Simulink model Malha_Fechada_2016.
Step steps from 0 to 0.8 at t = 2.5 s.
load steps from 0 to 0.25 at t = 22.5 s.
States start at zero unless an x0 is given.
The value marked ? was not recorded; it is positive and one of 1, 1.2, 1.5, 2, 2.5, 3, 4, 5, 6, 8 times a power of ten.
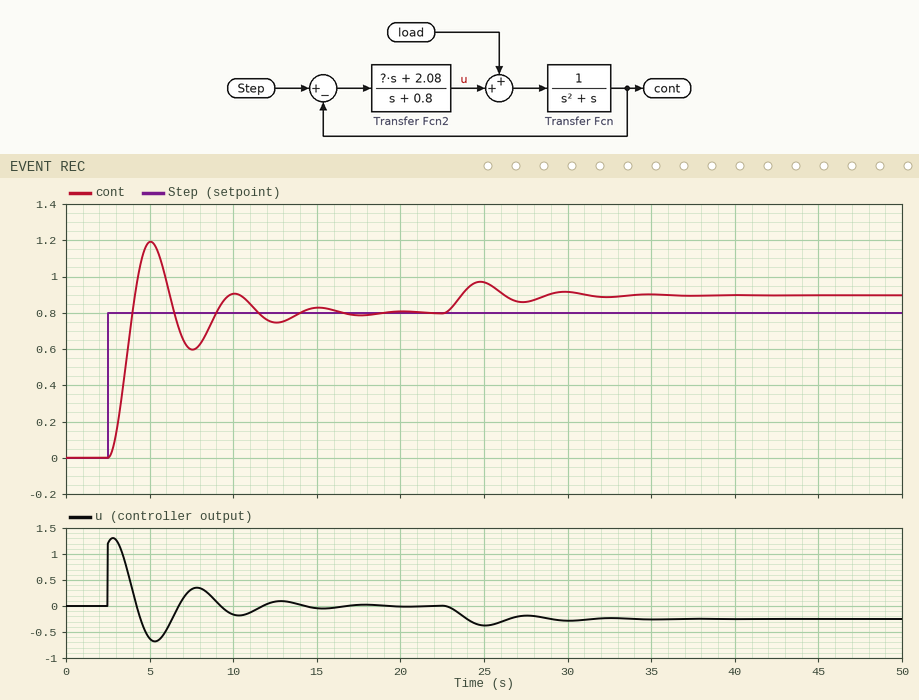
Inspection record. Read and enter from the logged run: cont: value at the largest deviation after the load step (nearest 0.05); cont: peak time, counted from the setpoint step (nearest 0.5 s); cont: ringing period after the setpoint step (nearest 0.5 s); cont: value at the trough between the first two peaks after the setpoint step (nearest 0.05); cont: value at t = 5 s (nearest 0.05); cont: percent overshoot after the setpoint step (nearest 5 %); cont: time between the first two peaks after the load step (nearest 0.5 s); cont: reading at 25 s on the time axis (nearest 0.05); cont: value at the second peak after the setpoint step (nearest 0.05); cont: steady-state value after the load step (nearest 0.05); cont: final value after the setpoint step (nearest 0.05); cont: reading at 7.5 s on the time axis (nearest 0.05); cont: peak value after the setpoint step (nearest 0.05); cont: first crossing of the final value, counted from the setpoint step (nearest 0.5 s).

0.95
2.5 s
5.0 s
0.60
1.20
50 %
5.0 s
0.95
0.90
0.90
0.80
0.60
1.20
1.5 s
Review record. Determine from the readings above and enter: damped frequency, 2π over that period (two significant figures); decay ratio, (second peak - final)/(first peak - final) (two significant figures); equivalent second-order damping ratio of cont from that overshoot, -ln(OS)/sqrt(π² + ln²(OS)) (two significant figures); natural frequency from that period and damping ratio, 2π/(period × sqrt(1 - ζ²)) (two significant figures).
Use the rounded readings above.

1.3 rad/s
0.25
0.22
1.3 rad/s
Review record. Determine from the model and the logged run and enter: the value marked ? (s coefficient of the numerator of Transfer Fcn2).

1.5
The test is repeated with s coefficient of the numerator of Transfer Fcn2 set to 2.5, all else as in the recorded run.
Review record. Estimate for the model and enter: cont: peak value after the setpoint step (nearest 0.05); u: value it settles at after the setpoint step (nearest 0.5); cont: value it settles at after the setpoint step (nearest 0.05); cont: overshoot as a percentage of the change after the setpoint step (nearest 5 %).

1.10
0.0
0.80
35 %
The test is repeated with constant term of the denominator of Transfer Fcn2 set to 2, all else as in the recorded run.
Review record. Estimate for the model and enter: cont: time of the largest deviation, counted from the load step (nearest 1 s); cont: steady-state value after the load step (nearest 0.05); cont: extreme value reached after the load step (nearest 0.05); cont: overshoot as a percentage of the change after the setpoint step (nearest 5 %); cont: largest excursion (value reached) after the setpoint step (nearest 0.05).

4 s
1.05
1.05
10 %
0.90
